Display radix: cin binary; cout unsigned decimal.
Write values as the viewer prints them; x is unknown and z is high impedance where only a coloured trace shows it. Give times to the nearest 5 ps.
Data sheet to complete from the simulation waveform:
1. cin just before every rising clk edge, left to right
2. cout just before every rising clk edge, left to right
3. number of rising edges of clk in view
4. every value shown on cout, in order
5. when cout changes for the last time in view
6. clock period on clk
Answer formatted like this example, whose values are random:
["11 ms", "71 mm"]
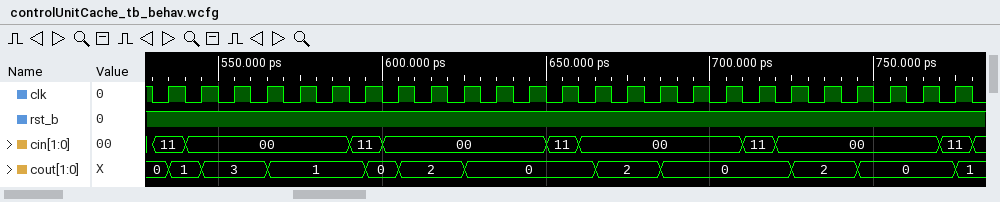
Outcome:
["11, 00, 00, 00, 00, 00, 11, 00, 00, 00, 00, 00, 11, 00, 00, 00, 00, 00, 11, 00, 00, 00, 00, 00, 11", "0, 1, 3, 3, 1, 1, 1, 0, 2, 2, 0, 0, 0, 0, 2, 2, 0, 0, 0, 0, 2, 2, 0, 0, 0", "25", "0, 1, 3, 1, 0, 2, 0, 2, 0, 2, 0, 1", "775 ps", "10 ps"]
